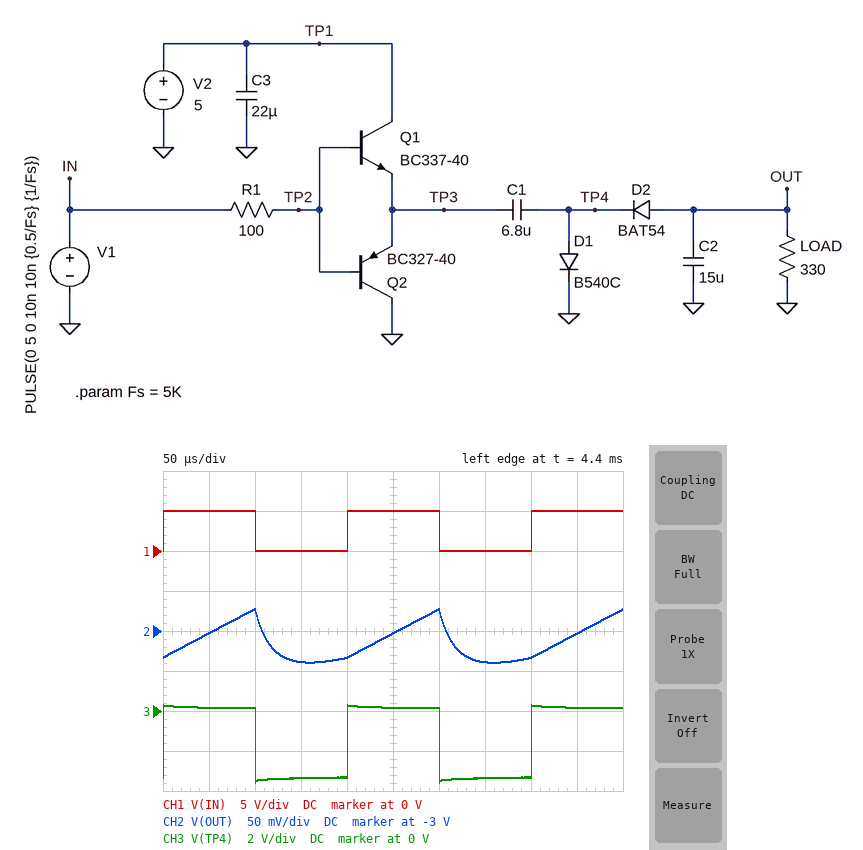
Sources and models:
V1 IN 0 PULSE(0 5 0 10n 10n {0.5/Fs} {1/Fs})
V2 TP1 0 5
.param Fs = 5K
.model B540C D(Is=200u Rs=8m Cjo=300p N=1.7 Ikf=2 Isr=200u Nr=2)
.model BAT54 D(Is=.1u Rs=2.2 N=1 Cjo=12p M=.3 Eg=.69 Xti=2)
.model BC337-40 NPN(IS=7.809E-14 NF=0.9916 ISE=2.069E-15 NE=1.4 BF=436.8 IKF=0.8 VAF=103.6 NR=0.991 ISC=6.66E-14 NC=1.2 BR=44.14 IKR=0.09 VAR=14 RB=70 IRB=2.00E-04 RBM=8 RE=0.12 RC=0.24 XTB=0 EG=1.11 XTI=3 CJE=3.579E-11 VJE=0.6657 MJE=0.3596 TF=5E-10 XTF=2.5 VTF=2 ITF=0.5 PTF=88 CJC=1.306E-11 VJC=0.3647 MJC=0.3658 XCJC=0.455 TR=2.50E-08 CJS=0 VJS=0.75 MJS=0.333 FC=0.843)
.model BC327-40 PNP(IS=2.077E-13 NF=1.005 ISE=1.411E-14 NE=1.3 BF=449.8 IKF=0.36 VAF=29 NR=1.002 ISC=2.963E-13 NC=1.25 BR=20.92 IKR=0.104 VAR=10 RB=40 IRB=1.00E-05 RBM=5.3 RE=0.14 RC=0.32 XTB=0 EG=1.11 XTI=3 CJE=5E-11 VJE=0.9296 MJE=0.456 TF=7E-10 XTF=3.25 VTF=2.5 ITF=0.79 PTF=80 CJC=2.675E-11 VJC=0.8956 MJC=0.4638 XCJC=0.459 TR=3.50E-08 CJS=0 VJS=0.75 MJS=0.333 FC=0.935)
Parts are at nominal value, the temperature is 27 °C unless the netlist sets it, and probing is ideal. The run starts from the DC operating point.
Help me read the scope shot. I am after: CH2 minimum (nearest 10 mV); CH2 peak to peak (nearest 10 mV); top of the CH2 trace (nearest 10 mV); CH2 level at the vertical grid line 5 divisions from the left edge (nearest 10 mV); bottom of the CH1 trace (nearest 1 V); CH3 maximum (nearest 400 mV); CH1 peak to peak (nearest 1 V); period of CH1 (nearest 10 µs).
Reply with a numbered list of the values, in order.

1. -3.04 V
2. 70 mV
3. -2.97 V
4. -3.00 V
5. 0 V
6. 400 mV
7. 5 V
8. 200 µs
